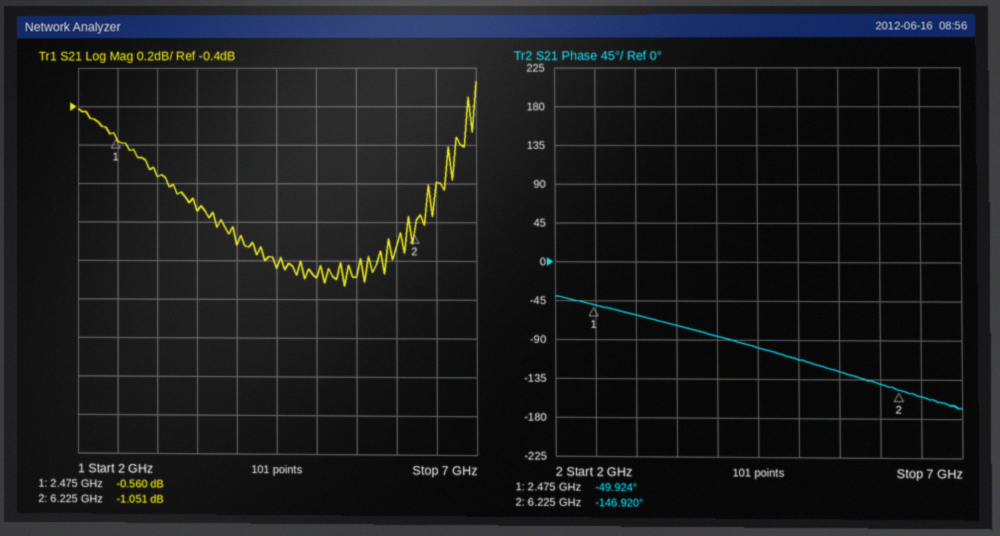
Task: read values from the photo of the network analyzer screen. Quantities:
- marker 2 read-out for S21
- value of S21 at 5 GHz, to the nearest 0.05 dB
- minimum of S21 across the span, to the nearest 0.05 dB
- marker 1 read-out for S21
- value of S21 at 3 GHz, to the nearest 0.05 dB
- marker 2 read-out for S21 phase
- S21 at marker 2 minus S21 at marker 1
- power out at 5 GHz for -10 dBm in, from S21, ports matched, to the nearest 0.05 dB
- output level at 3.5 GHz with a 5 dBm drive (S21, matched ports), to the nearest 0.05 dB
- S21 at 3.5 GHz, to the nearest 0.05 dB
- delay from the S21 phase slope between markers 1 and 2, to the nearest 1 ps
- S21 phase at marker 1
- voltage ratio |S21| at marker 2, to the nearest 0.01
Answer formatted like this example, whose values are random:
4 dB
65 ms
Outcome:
-1.051 dB
-1.30 dB
-1.35 dB
-0.560 dB
-0.75 dB
-146.920°
-0.491 dB
-11.30 dBm
4.05 dBm
-0.95 dB
72 ps
-49.924°
0.89
